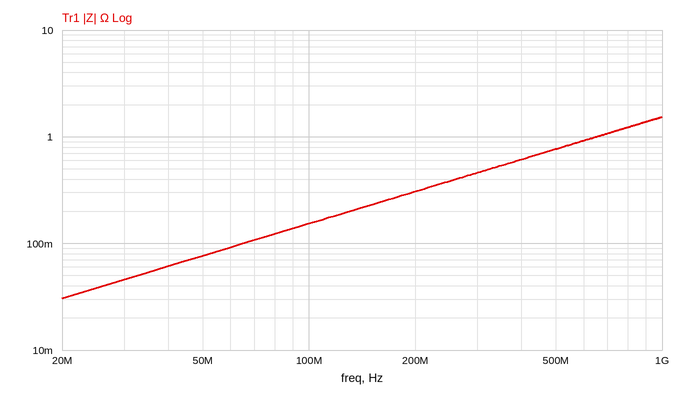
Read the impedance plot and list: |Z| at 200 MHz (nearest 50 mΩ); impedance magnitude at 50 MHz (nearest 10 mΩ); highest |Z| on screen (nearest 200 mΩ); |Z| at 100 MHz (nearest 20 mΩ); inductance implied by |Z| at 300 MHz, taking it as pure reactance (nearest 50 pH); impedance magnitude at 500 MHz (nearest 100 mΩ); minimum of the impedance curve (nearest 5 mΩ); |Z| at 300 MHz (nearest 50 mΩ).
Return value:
300 mΩ
80 mΩ
1.6 Ω
160 mΩ
250 pH
800 mΩ
30 mΩ
450 mΩ
